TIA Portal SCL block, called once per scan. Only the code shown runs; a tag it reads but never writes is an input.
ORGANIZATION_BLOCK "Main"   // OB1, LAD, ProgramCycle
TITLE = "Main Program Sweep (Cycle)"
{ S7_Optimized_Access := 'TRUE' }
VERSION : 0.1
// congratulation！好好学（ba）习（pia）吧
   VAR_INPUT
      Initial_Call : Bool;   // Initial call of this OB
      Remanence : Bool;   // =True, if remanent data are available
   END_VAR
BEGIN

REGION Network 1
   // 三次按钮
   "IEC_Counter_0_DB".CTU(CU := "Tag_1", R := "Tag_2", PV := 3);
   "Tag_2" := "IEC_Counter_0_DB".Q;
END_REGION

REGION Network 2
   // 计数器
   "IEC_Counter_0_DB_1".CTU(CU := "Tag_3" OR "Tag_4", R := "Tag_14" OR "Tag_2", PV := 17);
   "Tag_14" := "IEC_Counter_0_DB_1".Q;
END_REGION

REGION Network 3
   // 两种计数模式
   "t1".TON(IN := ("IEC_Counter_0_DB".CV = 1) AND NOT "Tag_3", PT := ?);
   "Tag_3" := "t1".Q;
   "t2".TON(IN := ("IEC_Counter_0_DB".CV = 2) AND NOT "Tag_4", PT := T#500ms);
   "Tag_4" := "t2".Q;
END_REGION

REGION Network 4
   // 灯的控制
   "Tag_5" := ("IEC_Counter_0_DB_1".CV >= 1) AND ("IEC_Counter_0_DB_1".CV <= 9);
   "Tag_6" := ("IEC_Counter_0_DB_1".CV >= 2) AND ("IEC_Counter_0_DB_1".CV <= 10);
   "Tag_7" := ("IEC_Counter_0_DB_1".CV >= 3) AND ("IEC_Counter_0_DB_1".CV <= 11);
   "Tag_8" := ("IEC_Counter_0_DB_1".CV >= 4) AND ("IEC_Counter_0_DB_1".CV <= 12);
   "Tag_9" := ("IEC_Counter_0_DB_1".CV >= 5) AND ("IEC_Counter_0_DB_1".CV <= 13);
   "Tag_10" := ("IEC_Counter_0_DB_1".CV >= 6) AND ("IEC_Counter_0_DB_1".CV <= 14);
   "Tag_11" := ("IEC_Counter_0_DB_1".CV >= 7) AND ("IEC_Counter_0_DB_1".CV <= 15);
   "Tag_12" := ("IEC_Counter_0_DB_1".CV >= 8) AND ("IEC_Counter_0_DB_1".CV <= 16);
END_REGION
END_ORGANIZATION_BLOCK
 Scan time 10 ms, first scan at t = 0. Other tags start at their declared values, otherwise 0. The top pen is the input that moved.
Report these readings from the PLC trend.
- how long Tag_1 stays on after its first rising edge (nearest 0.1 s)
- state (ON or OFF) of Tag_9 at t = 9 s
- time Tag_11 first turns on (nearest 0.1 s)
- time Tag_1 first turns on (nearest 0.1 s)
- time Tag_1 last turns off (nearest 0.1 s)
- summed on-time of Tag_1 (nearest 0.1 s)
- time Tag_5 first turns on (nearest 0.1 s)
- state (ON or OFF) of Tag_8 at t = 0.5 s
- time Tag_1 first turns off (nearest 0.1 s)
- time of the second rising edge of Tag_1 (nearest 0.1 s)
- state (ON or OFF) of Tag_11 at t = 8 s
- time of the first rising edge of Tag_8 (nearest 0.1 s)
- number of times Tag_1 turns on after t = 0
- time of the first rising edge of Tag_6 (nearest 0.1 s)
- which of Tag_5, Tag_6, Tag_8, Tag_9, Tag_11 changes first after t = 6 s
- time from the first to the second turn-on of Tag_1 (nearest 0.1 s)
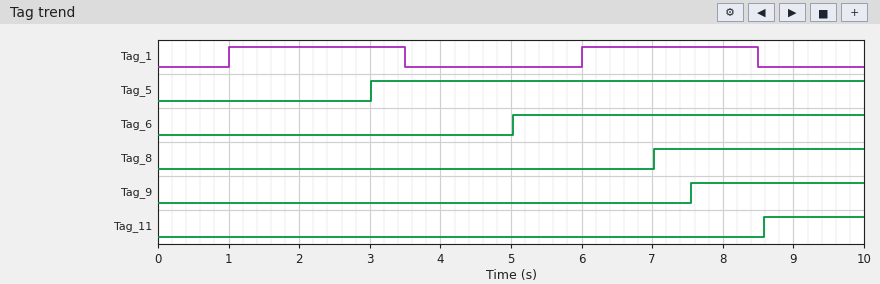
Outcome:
2.5 s
ON
8.6 s
1.0 s
8.5 s
5.0 s
3.0 s
OFF
3.5 s
6.0 s
OFF
7.0 s
2
5.0 s
Tag_8
5.0 s
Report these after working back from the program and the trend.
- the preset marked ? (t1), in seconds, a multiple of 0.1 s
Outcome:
2.0 s
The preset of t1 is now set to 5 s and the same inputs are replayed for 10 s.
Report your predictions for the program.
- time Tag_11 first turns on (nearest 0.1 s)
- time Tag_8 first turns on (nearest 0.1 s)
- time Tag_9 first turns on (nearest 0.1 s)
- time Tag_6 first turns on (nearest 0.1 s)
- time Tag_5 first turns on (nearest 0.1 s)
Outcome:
9.6 s
8.1 s
8.6 s
7.0 s
6.5 s
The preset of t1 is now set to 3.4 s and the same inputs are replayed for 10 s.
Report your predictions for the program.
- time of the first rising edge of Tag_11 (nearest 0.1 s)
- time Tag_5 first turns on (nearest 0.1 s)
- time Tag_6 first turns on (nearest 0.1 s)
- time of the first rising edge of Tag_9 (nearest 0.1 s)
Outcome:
9.1 s
4.4 s
6.5 s
8.1 s
